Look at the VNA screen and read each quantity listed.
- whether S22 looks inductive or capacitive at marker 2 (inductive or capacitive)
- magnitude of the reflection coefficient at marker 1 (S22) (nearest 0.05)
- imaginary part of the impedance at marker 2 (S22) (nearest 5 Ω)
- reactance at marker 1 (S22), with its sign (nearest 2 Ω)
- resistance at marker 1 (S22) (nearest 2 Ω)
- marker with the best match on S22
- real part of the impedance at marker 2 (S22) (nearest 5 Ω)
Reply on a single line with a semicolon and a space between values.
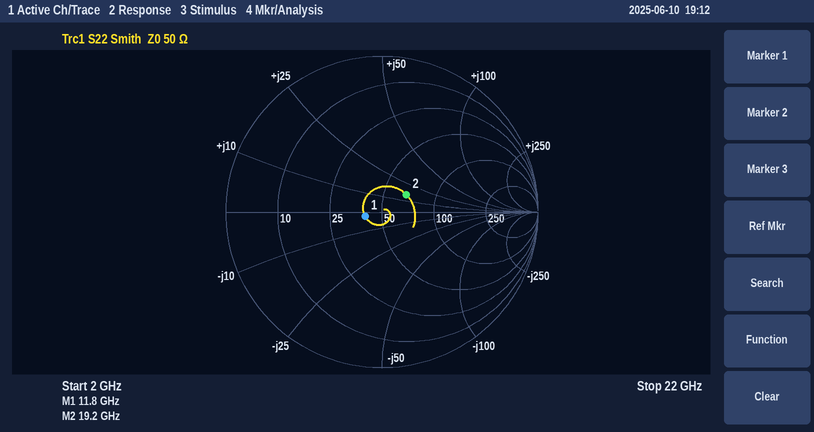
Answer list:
inductive; 0.10; +15 Ω; -2 Ω; 40 Ω; marker 1; 65 Ω
